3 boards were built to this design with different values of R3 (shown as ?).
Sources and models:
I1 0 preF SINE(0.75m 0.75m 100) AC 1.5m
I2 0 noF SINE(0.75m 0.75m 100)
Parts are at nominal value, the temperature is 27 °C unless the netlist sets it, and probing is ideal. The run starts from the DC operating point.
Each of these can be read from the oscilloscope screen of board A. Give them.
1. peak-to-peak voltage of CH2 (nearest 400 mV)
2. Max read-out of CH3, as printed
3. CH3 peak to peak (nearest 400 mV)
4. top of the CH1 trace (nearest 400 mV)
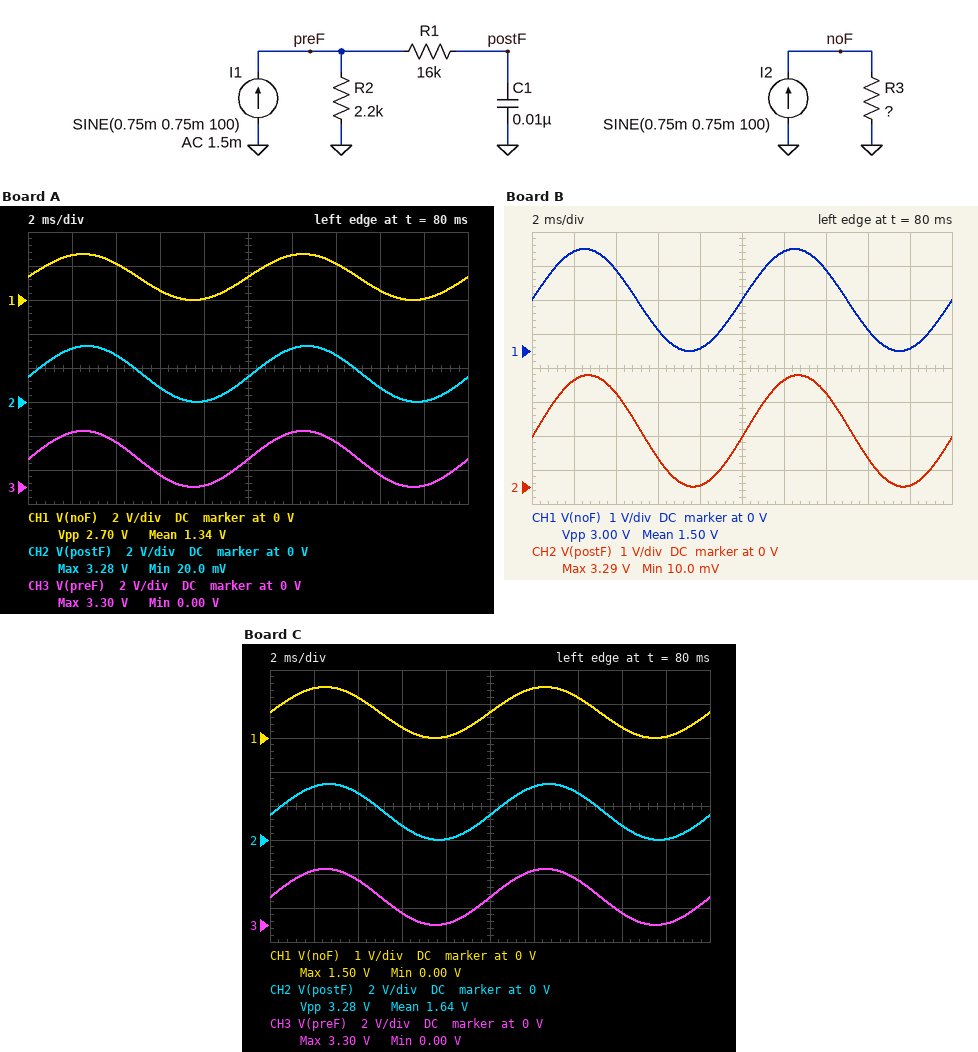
3.2 V
3.30 V
3.2 V
2.8 V
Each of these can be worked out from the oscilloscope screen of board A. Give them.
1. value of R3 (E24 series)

1.8 kΩ
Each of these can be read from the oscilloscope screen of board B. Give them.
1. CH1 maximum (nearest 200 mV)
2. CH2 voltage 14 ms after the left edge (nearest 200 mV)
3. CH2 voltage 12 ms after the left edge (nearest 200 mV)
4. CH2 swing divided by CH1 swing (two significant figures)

3.0 V
2.8 V
3.2 V
1.1
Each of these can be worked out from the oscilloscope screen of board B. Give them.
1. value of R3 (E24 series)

2 kΩ
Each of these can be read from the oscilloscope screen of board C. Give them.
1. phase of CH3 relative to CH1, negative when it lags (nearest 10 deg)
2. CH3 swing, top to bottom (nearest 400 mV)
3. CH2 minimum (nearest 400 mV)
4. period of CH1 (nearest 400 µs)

0 deg
3.2 V
0 V
10.0 ms
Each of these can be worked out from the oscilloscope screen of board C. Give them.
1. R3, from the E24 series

1 kΩ
